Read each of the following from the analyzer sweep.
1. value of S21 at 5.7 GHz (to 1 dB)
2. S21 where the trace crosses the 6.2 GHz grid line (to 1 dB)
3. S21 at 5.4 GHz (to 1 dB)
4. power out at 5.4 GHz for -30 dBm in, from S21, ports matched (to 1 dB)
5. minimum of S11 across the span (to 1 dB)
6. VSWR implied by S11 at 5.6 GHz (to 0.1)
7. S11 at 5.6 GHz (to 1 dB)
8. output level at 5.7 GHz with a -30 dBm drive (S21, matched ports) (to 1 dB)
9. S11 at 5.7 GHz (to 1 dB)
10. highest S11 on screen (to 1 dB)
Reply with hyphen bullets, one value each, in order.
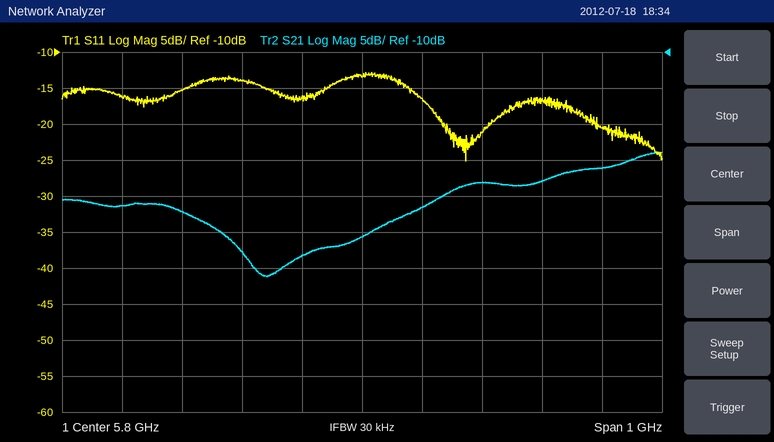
- -38 dB
- -26 dB
- -31 dB
- -61 dBm
- -25 dB
- 1.5
- -14 dB
- -68 dBm
- -16 dB
- -13 dB
